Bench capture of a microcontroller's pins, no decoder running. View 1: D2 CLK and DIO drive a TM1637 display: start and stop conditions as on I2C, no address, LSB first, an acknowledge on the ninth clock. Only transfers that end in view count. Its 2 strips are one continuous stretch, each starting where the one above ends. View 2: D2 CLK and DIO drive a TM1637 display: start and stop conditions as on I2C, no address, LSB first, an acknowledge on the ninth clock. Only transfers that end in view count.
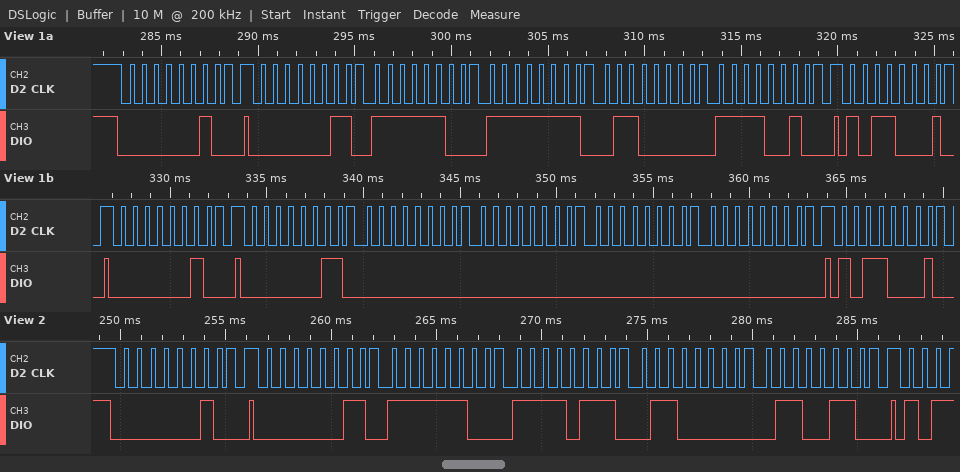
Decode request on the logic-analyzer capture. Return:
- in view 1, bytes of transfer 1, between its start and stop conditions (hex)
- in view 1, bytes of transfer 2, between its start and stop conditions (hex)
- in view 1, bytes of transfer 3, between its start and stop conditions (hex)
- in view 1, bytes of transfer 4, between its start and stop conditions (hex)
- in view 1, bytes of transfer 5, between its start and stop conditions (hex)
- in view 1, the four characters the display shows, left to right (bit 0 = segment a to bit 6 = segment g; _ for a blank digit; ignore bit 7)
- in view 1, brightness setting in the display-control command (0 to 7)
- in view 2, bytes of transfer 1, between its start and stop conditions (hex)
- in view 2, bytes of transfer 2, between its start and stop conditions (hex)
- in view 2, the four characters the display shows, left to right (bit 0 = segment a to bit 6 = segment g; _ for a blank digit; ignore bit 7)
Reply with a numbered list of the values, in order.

1. 40
2. C0 3F FF 06 4F
3. 8D
4. 40
5. C0 00 00 00 00
6. ____
7. 5
8. 40
9. C0 3F EF 06 66
10. 0914
